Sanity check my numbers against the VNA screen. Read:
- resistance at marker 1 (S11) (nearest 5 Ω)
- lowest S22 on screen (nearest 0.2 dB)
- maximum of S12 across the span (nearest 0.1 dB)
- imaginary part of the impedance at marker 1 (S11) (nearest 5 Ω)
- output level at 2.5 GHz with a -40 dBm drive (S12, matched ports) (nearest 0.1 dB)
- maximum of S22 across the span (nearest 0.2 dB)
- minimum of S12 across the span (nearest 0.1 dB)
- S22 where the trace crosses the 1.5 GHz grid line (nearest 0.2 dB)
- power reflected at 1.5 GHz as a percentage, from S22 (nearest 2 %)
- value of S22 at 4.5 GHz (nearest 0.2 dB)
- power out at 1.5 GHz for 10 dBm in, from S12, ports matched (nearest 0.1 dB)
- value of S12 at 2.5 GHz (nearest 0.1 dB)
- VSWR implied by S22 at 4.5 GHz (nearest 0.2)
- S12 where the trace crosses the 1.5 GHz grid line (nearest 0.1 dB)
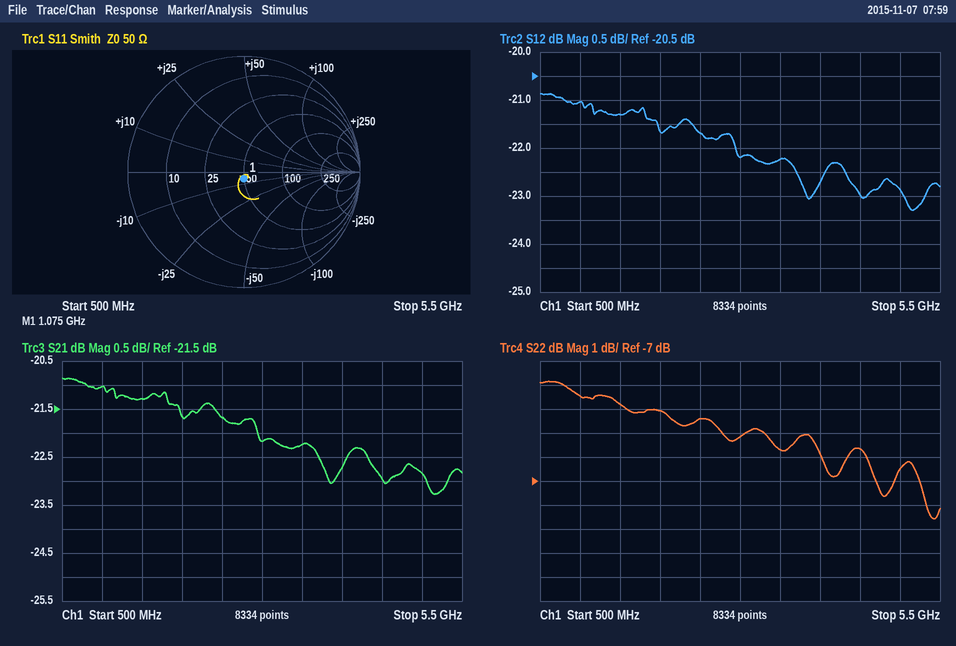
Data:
50 Ω
-8.6 dB
-20.9 dB
-5 Ω
-61.7 dBm
-2.8 dB
-23.3 dB
-3.8 dB
42 %
-5.6 dB
-11.3 dBm
-21.7 dB
3.2
-21.3 dB
